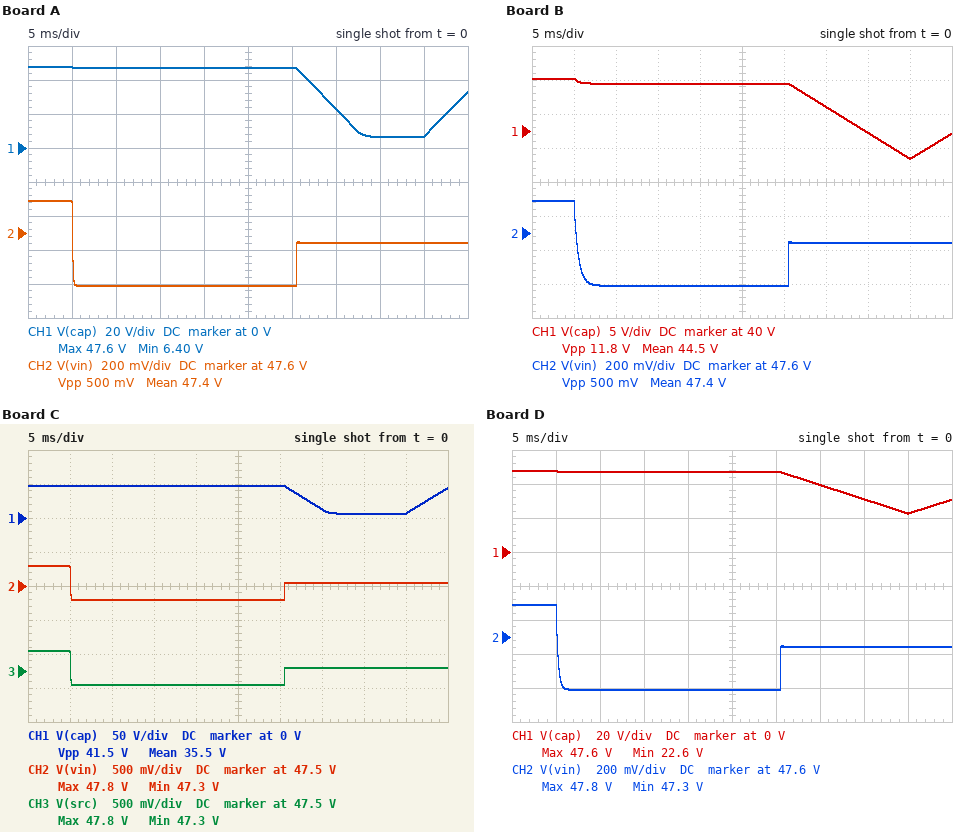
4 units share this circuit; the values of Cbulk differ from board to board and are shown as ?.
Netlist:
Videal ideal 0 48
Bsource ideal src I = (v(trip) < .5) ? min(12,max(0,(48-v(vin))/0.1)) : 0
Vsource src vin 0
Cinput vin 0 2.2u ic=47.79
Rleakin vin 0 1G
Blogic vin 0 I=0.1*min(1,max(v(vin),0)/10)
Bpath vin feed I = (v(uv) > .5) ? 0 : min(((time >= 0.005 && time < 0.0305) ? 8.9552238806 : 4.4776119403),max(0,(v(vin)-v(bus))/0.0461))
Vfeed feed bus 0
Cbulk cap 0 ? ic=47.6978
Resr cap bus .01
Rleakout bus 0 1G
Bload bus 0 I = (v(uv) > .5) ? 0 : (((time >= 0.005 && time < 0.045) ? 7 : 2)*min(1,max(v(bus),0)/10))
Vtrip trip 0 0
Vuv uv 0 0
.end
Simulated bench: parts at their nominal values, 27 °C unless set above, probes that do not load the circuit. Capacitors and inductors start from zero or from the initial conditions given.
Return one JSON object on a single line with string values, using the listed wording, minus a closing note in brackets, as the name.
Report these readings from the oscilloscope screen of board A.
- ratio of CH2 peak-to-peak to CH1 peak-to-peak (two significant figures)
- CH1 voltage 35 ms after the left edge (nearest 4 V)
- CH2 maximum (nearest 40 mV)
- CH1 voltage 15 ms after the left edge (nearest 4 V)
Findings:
{"ratio of CH2 peak-to-peak to CH1 peak-to-peak": "0.012", "CH1 voltage 35 ms after the left edge": "24 V", "CH2 maximum": "47.80 V", "CH1 voltage 15 ms after the left edge": "48 V"}
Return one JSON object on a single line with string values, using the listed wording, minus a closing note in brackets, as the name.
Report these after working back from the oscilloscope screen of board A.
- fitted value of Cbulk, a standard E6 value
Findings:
{"fitted value of Cbulk, a standard E6 value": "470 µF"}
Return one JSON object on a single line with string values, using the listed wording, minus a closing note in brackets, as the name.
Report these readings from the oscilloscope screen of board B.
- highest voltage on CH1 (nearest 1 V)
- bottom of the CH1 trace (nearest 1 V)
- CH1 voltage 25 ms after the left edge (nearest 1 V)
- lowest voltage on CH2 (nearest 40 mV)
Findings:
{"highest voltage on CH1": "48 V", "bottom of the CH1 trace": "36 V", "CH1 voltage 25 ms after the left edge": "47 V", "lowest voltage on CH2": "47.28 V"}
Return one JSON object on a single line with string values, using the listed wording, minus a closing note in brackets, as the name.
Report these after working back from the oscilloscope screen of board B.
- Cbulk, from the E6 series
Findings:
{"Cbulk, from the E6 series": "3.3 mF"}
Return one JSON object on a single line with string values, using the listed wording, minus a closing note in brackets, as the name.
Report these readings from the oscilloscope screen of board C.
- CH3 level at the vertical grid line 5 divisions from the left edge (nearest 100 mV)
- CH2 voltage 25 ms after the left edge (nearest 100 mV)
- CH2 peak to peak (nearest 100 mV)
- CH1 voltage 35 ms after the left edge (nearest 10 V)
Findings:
{"CH3 level at the vertical grid line 5 divisions from the left edge": "47.3 V", "CH2 voltage 25 ms after the left edge": "47.3 V", "CH2 peak to peak": "500 mV", "CH1 voltage 35 ms after the left edge": "10 V"}
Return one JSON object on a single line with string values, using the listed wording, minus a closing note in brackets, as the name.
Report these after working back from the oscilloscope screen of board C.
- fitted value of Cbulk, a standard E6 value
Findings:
{"fitted value of Cbulk, a standard E6 value": "330 µF"}
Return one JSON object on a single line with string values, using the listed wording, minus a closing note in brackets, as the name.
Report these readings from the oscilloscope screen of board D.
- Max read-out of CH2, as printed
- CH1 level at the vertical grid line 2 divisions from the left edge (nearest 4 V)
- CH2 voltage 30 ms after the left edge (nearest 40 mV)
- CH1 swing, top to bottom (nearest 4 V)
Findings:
{"Max read-out of CH2, as printed": "47.8 V", "CH1 level at the vertical grid line 2 divisions from the left edge": "48 V", "CH2 voltage 30 ms after the left edge": "47.28 V", "CH1 swing, top to bottom": "24 V"}
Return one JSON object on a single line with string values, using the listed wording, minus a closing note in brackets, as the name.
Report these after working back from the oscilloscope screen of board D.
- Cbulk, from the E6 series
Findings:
{"Cbulk, from the E6 series": "1.5 mF"}
